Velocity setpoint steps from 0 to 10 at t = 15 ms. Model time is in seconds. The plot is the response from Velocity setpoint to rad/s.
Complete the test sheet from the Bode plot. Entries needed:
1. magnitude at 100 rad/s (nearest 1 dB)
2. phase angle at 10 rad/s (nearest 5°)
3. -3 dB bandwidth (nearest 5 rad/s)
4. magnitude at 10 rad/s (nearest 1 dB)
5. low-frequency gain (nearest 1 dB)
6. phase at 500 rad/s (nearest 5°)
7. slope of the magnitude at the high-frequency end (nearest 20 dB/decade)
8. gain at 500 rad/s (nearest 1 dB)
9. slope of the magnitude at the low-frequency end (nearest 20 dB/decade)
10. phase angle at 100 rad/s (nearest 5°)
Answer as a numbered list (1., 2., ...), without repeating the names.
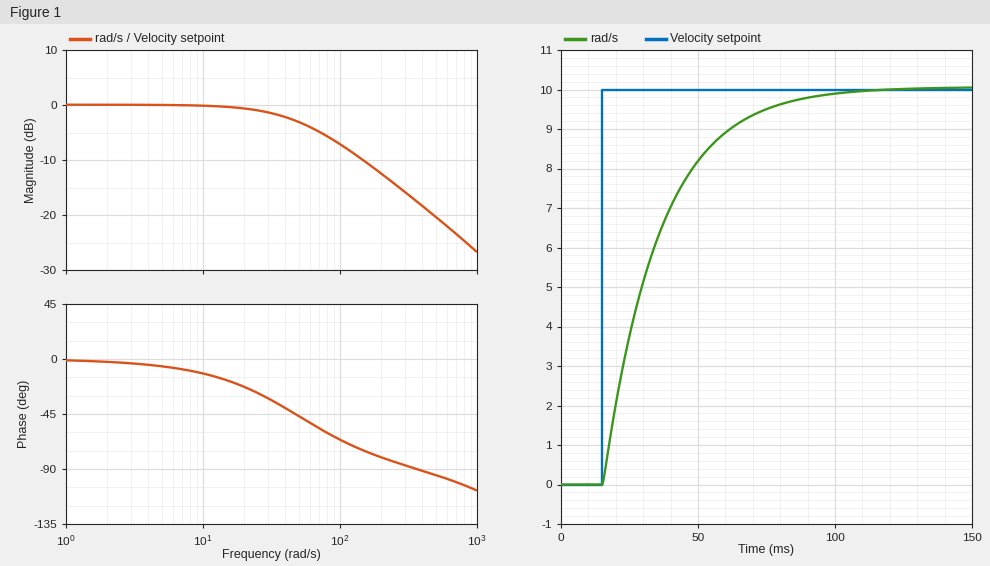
1. -7 dB
2. -10°
3. 50 rad/s
4. 0 dB
5. 0 dB
6. -95°
7. -20 dB/decade
8. -20 dB
9. 0 dB/decade
10. -65°
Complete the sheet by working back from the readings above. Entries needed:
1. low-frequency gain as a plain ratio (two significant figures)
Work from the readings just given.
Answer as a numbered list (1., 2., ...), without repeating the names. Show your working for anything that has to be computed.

1. 10^(0 / 20) = 1.0
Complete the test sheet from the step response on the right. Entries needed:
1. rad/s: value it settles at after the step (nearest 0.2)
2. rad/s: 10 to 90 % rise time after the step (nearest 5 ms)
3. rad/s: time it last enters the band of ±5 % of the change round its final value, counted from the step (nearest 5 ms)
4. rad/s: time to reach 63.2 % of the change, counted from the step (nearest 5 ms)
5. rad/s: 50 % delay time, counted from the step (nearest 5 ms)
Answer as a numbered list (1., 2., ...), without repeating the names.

1. 10.0
2. 45 ms
3. 60 ms
4. 20 ms
5. 15 ms
